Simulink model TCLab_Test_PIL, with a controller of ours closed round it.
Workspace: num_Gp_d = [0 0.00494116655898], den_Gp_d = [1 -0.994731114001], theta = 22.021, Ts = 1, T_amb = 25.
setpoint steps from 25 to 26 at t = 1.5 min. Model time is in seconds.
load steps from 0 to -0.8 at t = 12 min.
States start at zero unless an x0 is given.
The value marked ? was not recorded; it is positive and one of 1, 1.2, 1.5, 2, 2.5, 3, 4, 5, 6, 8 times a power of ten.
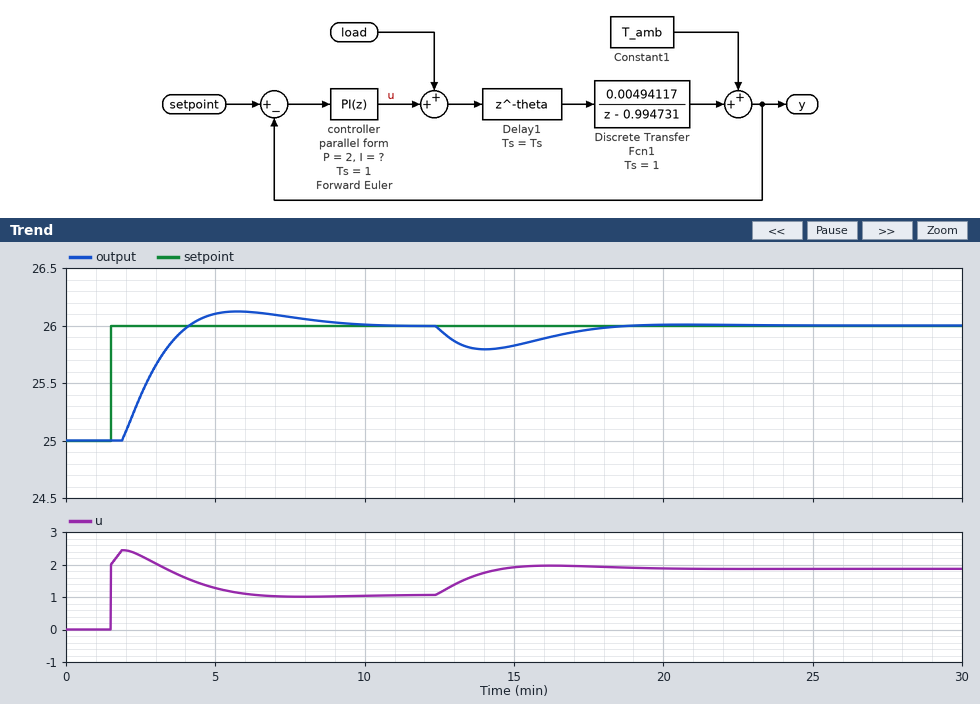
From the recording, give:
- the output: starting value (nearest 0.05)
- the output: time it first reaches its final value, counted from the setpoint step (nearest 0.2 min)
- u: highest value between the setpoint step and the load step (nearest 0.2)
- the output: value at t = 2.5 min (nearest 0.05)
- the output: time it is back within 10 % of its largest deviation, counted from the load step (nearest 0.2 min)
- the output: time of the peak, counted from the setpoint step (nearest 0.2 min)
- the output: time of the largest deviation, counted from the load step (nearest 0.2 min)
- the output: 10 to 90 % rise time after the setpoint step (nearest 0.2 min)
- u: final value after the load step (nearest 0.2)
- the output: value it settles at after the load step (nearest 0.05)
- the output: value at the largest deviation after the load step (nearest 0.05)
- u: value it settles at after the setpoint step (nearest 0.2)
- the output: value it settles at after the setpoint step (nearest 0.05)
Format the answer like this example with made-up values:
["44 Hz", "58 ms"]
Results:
["25.00", "2.6 min", "2.4", "25.40", "6.0 min", "4.2 min", "2.0 min", "1.6 min", "1.8", "26.00", "25.80", "1.0", "26.00"]
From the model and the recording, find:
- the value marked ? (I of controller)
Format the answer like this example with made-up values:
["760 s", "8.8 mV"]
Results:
["0.02"]
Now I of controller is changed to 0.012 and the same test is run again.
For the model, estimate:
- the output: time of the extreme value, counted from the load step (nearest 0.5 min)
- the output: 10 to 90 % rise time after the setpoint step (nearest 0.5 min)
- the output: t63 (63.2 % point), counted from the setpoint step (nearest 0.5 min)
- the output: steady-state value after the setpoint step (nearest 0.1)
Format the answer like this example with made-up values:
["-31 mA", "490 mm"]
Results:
["2.5 min", "2.5 min", "1.5 min", "26.0"]
